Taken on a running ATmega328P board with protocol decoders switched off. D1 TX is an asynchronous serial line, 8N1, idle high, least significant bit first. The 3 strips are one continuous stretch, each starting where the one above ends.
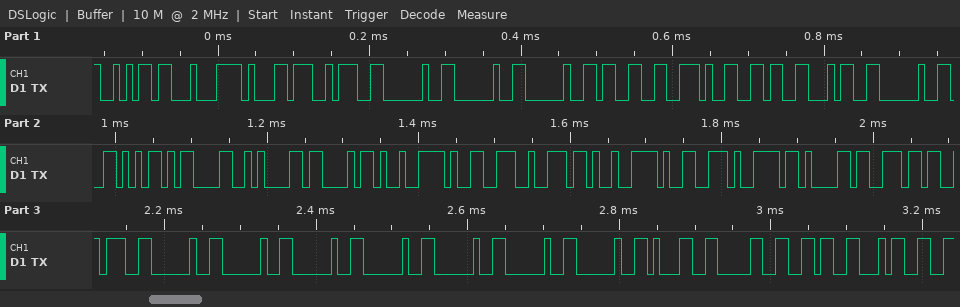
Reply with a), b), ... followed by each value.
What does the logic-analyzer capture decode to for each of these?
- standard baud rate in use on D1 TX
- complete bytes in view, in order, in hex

a) 115200 baud
b) 6A C4 B1 3A 20 20 20 33 2E 36 34 20 56 0D 0A 43 C9 99 72 C9 99 79 61 6E 3A 20 20 20 20 20 20 20 31 30 36 34
